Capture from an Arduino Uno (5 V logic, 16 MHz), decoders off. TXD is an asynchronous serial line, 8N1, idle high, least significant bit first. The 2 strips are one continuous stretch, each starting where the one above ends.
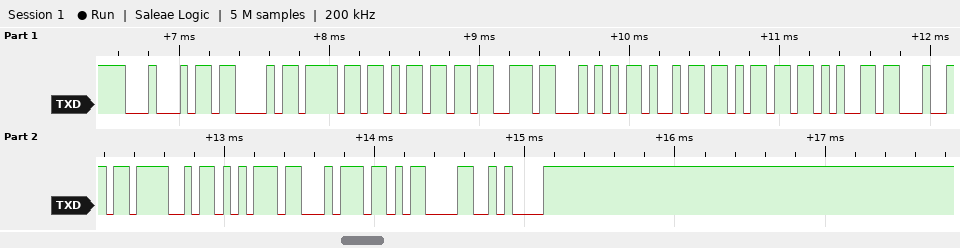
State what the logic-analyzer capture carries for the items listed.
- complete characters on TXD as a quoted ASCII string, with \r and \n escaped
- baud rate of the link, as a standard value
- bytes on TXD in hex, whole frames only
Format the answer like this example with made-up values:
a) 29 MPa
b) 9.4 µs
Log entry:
a) "DComsTimedOut\r\n"
b) 19200 baud
c) 44 43 6F 6D 73 54 69 6D 65 64 4F 75 74 0D 0A
